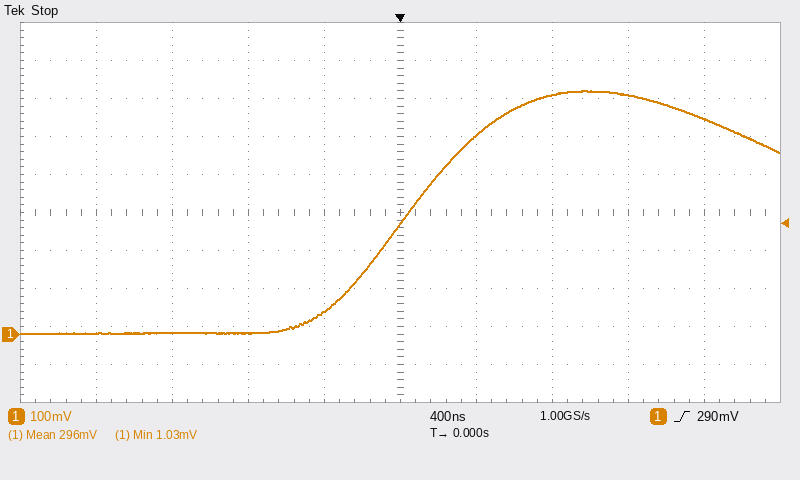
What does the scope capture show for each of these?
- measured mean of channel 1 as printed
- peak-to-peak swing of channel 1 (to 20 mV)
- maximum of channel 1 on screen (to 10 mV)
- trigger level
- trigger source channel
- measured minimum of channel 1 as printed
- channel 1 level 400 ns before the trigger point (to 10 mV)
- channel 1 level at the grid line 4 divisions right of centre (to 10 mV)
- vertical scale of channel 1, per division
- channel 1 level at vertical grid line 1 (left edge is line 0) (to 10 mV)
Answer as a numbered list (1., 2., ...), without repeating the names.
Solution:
1. 296 mV
2. 640 mV
3. 640 mV
4. 290 mV
5. channel 1
6. 1.03 mV
7. 60 mV
8. 570 mV
9. 100 mV
10. 0 mV
